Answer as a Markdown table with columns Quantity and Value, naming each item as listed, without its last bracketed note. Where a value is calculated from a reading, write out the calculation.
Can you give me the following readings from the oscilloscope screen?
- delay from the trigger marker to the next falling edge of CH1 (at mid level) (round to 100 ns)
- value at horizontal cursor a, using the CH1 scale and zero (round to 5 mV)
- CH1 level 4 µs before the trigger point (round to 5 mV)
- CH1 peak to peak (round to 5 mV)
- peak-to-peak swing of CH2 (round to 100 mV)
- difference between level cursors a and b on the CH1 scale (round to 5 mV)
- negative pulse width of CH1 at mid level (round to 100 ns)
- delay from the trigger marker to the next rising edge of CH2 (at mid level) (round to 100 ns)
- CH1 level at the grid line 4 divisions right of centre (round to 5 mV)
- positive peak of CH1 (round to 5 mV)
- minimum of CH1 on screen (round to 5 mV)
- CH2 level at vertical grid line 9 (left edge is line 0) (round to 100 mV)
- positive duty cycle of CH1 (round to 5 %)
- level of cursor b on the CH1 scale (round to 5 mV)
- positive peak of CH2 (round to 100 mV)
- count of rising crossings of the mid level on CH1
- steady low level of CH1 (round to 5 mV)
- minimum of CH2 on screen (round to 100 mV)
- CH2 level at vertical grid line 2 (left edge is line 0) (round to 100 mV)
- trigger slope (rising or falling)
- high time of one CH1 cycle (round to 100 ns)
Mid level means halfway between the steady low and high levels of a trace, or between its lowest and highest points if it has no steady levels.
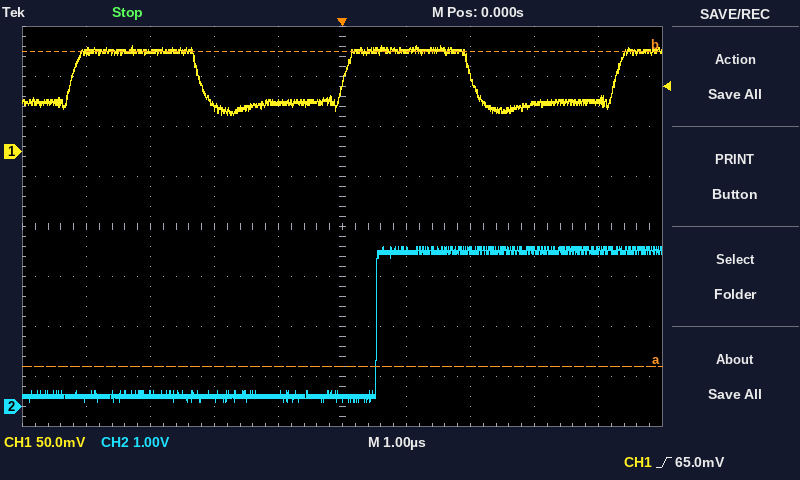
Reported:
| Quantity | Value |
|---|---|
| delay from the trigger marker to the next falling edge of CH1 (at mid level) | 2.0 µs |
| value at horizontal cursor a, using the CH1 scale and zero | -215 mV |
| CH1 level 4 µs before the trigger point | 100 mV |
| CH1 peak to peak | 105 mV − (35 mV) = 70 mV |
| peak-to-peak swing of CH2 | 3.2 V − (100 mV) = 3.1 V |
| difference between level cursors a and b on the CH1 scale | 315 mV |
| negative pulse width of CH1 at mid level | 2.3 µs |
| delay from the trigger marker to the next rising edge of CH2 (at mid level) | 500 ns |
| CH1 level at the grid line 4 divisions right of centre | 50 mV |
| positive peak of CH1 | 105 mV |
| minimum of CH1 on screen | 35 mV |
| CH2 level at vertical grid line 9 (left edge is line 0) | 3.1 V |
| positive duty cycle of CH1 | 45 % |
| level of cursor b on the CH1 scale | 100 mV |
| positive peak of CH2 | 3.2 V |
| count of rising crossings of the mid level on CH1 | 3 |
| steady low level of CH1 | 50 mV |
| minimum of CH2 on screen | 100 mV |
| CH2 level at vertical grid line 2 (left edge is line 0) | 200 mV |
| trigger slope | rising |
| high time of one CH1 cycle | 2.0 µs |
